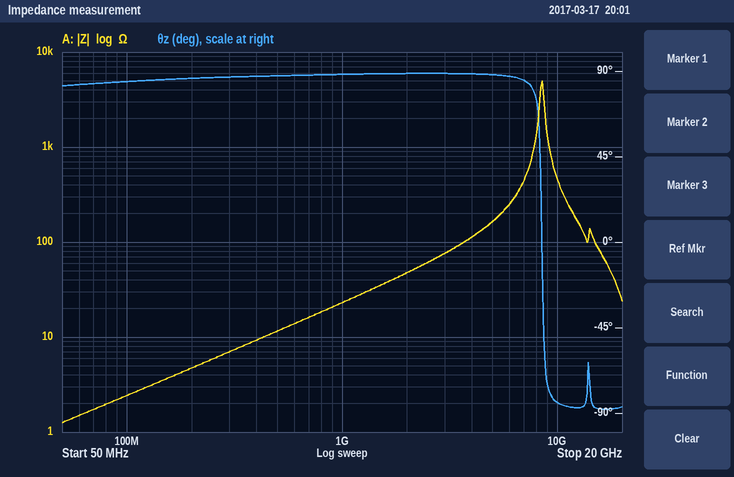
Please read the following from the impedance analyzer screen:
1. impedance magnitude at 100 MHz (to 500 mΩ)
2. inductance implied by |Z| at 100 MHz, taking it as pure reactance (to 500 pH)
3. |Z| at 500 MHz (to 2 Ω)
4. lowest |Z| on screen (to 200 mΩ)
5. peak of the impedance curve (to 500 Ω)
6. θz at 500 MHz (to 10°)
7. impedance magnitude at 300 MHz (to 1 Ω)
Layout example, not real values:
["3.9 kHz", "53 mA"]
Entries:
["2.5 Ω", "4.0 nH", "12 Ω", "1.2 Ω", "5.0 kΩ", "90°", "7 Ω"]
